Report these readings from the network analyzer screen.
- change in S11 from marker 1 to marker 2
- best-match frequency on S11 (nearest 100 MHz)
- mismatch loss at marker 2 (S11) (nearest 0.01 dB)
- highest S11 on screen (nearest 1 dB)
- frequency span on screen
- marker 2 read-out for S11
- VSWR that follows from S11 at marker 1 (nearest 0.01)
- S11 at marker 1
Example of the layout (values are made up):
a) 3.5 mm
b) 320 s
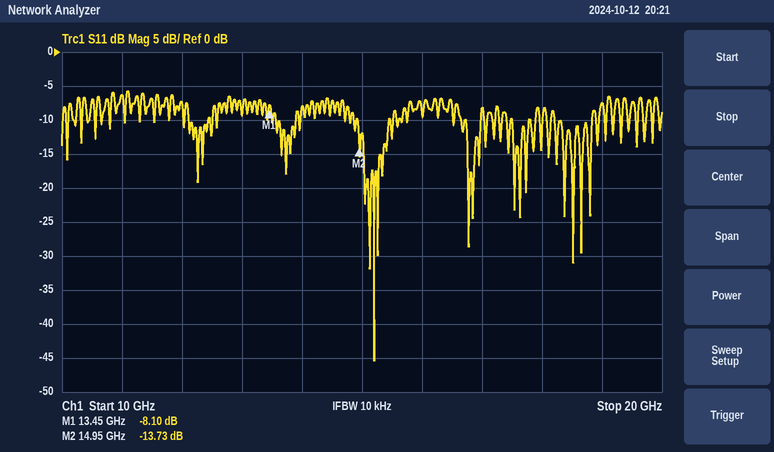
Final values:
a) -5.63 dB
b) 15.2 GHz
c) 0.19 dB
d) -6 dB
e) 10 GHz
f) -13.73 dB
g) 2.30
h) -8.10 dB
